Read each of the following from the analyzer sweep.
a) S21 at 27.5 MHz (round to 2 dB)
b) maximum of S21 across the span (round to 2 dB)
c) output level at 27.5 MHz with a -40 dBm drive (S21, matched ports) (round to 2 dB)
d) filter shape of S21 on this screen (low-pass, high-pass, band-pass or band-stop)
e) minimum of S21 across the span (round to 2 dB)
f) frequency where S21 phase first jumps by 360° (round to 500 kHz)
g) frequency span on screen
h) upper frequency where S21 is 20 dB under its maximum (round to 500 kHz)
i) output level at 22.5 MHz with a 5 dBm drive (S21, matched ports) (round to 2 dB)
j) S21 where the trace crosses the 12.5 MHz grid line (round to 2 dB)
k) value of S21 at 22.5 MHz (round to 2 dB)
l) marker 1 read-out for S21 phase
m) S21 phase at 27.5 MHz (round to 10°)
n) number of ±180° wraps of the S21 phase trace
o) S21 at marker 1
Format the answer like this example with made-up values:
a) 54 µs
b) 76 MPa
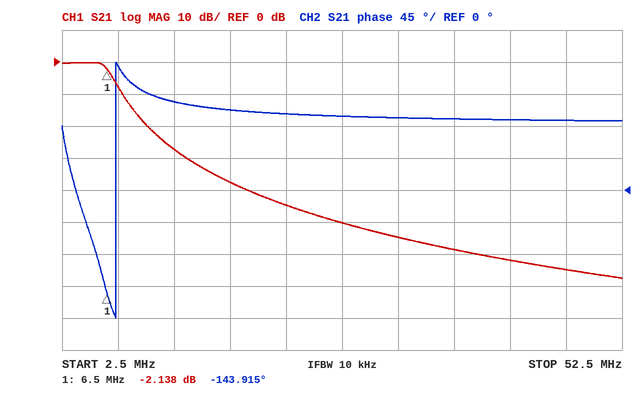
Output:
a) -50 dB
b) 0 dB
c) -90 dBm
d) low-pass
e) -68 dB
f) 7.5 MHz
g) 50 MHz
h) 10.0 MHz
i) -40 dBm
j) -28 dB
k) -44 dB
l) -143.915°
m) 100°
n) 1
o) -2.138 dB
